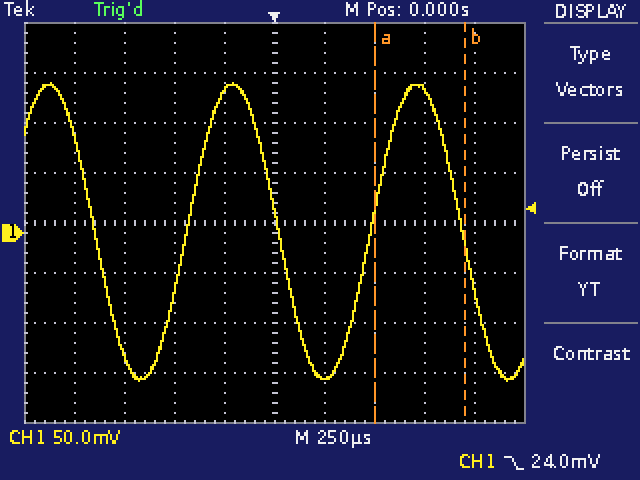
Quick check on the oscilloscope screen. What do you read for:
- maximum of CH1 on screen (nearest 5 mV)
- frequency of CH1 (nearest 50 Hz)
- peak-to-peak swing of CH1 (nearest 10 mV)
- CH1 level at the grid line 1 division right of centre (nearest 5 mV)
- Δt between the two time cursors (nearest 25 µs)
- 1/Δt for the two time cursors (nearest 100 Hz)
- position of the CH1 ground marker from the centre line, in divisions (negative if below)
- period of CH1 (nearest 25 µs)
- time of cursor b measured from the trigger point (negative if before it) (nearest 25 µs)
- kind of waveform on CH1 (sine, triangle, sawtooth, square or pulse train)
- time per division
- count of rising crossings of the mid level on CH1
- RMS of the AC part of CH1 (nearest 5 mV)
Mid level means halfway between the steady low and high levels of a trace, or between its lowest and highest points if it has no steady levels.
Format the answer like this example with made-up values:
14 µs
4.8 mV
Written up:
150 mV
1.10 kHz
300 mV
-145 mV
450 µs
2.2 kHz
-0.2 div
925 µs
+950 µs
sine
250 µs
2
105 mV
